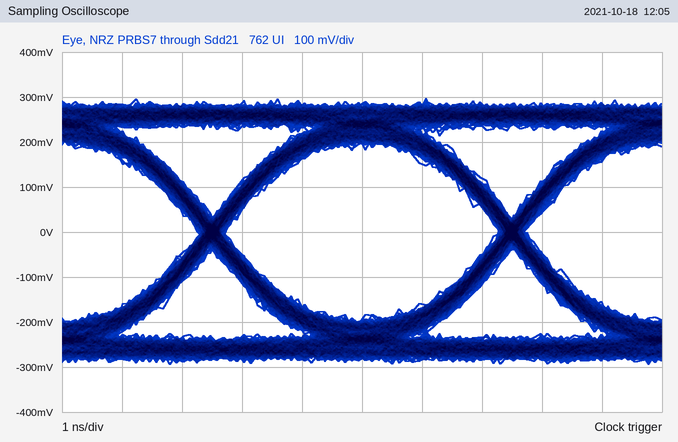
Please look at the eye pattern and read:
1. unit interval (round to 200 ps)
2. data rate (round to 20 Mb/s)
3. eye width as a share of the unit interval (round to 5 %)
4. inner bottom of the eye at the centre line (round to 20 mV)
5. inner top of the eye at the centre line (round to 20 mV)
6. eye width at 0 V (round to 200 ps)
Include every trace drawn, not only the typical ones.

5.0 ns
200 Mb/s
90 %
-200 mV
200 mV
4.6 ns
